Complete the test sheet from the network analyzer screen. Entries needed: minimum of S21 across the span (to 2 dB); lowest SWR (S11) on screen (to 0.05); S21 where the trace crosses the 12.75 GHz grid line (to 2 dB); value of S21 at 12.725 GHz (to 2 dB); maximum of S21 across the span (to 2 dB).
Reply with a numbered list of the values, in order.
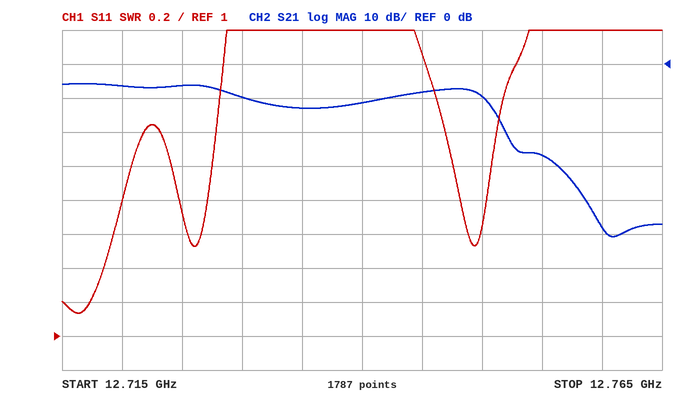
1. -50 dB
2. 1.15
3. -10 dB
4. -6 dB
5. -6 dB
